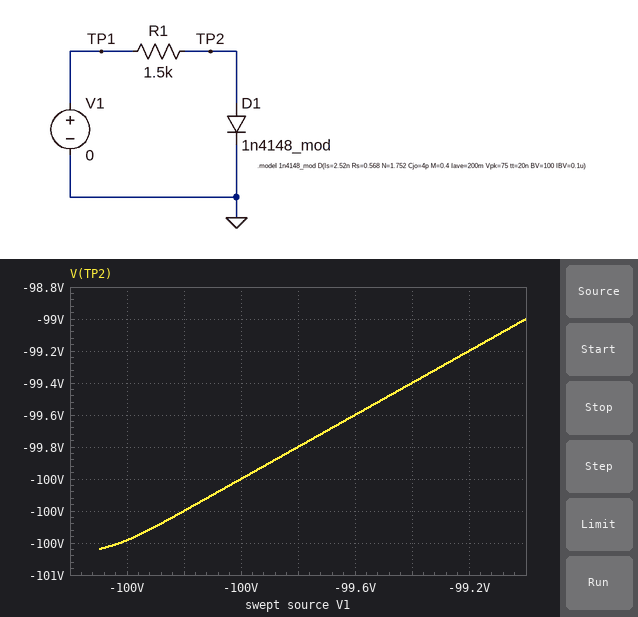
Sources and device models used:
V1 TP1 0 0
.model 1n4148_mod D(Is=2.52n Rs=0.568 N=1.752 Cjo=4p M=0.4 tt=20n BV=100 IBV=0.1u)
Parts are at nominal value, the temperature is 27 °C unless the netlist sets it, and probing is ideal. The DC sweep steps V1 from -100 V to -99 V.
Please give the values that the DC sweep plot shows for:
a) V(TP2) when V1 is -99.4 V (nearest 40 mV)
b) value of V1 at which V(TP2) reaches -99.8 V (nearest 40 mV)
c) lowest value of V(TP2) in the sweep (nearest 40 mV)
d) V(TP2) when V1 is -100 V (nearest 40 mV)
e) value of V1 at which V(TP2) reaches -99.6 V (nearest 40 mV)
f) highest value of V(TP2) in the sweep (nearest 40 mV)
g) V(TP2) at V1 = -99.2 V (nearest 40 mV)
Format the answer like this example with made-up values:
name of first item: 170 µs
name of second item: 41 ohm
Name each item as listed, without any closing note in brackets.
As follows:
V(TP2) when V1 is -99.4 V: -99.40 V
value of V1 at which V(TP2) reaches -99.8 V: -99.80 V
lowest value of V(TP2) in the sweep: -100.44 V
V(TP2) when V1 is -100 V: -100.00 V
value of V1 at which V(TP2) reaches -99.6 V: -99.60 V
highest value of V(TP2) in the sweep: -99.00 V
V(TP2) at V1 = -99.2 V: -99.20 V
